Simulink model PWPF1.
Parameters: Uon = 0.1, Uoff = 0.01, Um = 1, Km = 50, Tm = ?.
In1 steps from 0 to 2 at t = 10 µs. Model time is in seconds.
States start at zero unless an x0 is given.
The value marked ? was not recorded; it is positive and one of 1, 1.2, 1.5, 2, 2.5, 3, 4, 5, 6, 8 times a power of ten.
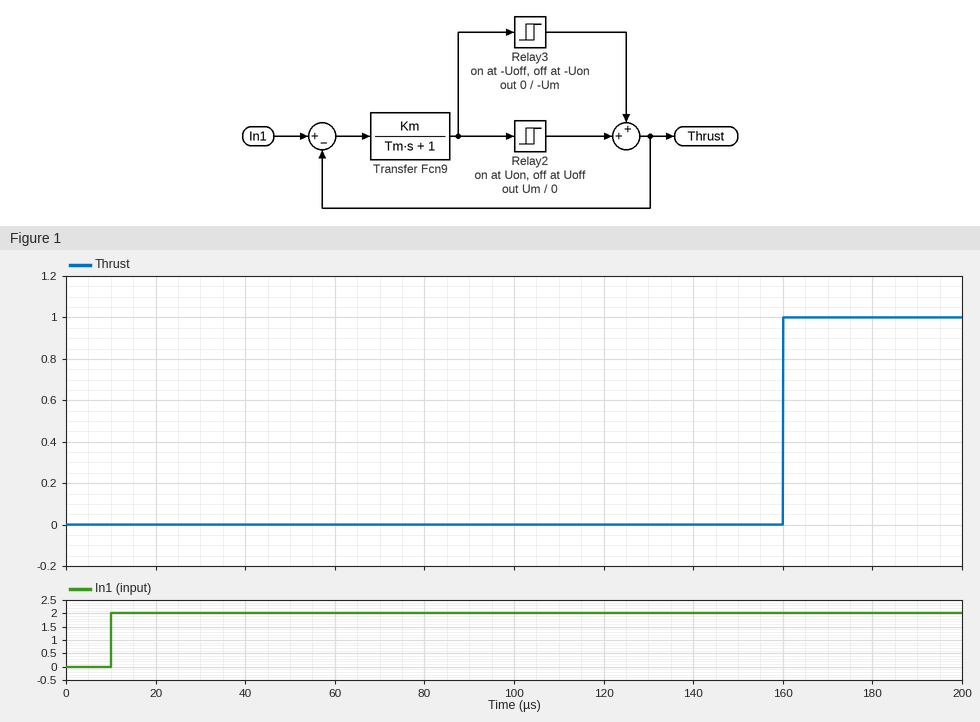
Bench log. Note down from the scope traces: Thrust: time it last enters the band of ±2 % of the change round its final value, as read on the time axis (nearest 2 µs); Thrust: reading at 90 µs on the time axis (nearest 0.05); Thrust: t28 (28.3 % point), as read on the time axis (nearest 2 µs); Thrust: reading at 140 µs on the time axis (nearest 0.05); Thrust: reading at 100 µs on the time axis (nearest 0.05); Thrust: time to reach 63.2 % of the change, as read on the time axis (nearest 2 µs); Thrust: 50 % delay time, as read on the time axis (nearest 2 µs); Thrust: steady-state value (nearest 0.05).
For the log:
160 µs
0.00
160 µs
0.00
0.00
160 µs
160 µs
1.00
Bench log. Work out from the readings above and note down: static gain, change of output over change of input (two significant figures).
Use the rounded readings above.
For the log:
0.50
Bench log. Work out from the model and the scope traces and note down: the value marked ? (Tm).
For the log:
0.15
